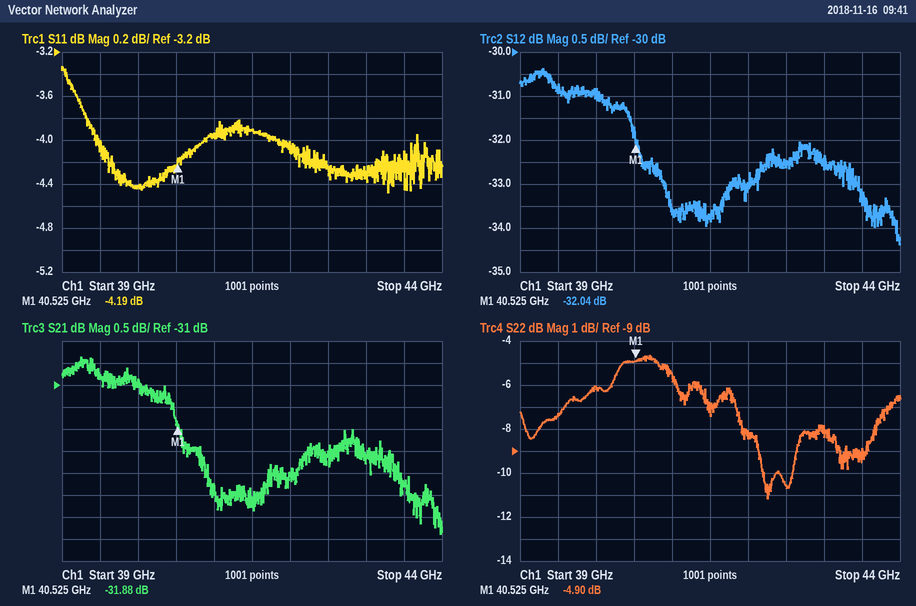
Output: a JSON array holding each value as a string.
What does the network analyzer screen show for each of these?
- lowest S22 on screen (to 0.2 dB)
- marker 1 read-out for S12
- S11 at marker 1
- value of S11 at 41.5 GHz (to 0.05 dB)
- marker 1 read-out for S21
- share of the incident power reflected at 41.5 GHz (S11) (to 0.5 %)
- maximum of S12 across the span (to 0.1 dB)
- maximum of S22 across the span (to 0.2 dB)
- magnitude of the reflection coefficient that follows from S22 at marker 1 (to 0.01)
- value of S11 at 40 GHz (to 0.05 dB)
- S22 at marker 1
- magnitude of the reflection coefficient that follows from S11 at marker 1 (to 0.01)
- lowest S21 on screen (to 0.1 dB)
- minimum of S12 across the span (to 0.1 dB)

["-11.2 dB", "-32.04 dB", "-4.19 dB", "-3.90 dB", "-31.88 dB", "40.5 %", "-30.4 dB", "-4.6 dB", "0.57", "-4.40 dB", "-4.90 dB", "0.62", "-34.4 dB", "-34.4 dB"]
